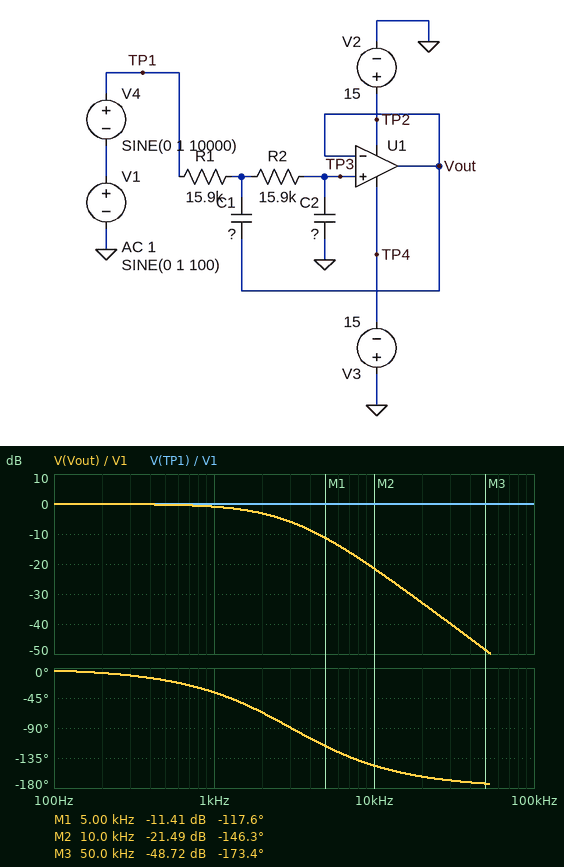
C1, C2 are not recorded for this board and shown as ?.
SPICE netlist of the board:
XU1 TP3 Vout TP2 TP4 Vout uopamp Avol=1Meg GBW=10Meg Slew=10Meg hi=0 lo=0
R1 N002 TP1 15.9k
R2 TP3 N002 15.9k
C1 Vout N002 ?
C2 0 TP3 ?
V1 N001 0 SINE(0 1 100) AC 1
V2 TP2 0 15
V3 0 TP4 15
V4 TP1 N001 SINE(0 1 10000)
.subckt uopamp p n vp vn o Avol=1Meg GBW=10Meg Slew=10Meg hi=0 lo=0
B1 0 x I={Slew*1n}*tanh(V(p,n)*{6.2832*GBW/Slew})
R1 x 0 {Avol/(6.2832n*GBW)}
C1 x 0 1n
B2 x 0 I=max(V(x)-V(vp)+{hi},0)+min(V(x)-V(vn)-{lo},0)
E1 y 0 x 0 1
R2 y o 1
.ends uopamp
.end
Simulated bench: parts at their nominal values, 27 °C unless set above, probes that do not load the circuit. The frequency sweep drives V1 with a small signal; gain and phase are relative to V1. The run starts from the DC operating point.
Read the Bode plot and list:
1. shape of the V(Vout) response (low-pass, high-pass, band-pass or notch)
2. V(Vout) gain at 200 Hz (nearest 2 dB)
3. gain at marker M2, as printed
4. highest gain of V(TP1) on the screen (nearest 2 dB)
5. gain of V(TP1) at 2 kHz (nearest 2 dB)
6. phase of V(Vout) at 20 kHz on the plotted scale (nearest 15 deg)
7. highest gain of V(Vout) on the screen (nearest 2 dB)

low-pass
0 dB
-21.49 dB
0 dB
0 dB
-165 deg
0 dB
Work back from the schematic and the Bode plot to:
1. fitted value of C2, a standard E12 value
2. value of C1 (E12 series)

3.3 nF
3.3 nF
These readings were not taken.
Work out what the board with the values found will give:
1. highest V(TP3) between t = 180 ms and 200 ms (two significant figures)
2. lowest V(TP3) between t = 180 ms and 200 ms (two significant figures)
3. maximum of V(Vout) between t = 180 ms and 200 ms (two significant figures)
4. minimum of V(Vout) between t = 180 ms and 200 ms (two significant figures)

1.1 V
-1.1 V
1.1 V
-1.1 V
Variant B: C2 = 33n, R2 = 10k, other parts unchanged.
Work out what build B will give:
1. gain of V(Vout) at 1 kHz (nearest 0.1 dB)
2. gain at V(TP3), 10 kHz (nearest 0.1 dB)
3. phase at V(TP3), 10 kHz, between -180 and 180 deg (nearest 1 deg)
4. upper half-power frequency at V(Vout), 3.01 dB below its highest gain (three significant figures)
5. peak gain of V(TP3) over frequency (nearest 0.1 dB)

-14.6 dB
-38.7 dB
-141 deg
191 Hz
0 dB
